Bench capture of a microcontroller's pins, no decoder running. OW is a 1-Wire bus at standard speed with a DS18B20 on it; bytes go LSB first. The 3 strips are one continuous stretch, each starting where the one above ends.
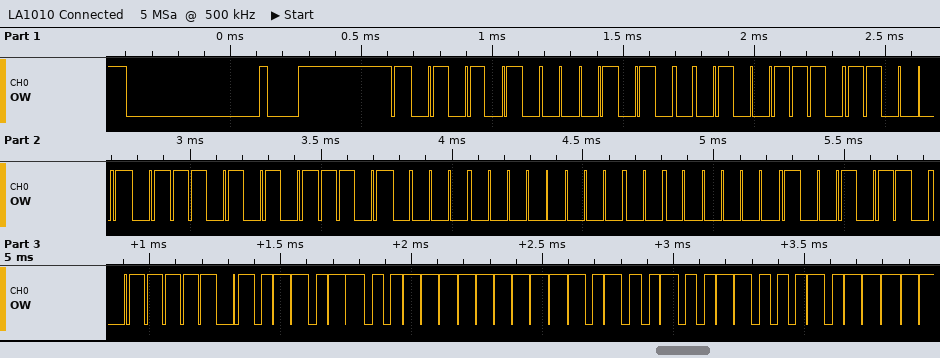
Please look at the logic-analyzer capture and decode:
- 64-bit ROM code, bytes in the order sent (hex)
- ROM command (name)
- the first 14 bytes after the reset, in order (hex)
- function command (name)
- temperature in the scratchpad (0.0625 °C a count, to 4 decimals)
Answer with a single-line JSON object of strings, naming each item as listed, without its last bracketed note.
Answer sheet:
{"64-bit ROM code, bytes in the order sent": "28 72 A3 AB 0B 00 00 69", "ROM command": "Match ROM", "the first 14 bytes after the reset, in order": "55 28 72 A3 AB 0B 00 00 69 BE 36 FF 4B 46", "function command": "Read Scratchpad", "temperature in the scratchpad": "-12.6250 °C"}
